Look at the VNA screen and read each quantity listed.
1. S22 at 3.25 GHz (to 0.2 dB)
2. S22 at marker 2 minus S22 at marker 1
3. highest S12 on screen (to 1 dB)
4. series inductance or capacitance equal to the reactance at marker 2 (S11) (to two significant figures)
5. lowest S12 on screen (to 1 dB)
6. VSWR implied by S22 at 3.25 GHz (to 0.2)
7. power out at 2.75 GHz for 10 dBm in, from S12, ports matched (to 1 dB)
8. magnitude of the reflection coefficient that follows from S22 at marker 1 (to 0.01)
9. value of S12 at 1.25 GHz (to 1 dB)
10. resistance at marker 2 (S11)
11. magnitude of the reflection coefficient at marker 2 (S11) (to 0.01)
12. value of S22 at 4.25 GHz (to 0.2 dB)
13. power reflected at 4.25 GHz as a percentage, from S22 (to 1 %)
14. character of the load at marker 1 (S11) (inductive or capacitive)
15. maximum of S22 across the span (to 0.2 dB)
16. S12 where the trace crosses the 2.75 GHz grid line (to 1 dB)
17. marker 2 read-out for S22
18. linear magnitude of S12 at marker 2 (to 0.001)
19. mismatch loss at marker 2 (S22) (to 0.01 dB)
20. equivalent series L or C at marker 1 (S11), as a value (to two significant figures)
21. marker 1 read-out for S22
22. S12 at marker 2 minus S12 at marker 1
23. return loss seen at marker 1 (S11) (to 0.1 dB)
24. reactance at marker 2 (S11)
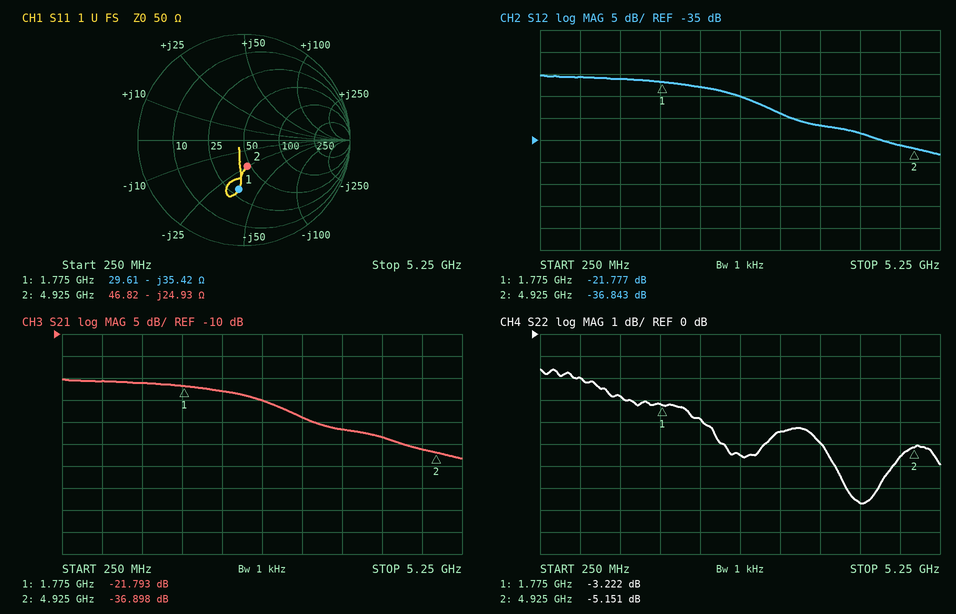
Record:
-4.4 dB
-1.929 dB
-20 dB
1.3 pF
-38 dB
4.0
-15 dBm
0.69
-21 dB
46.82 Ω
0.25
-7.6 dB
17 %
capacitive
-1.6 dB
-25 dB
-5.151 dB
0.014
1.58 dB
2.5 pF
-3.222 dB
-15.066 dB
6.6 dB
-24.93 Ω
